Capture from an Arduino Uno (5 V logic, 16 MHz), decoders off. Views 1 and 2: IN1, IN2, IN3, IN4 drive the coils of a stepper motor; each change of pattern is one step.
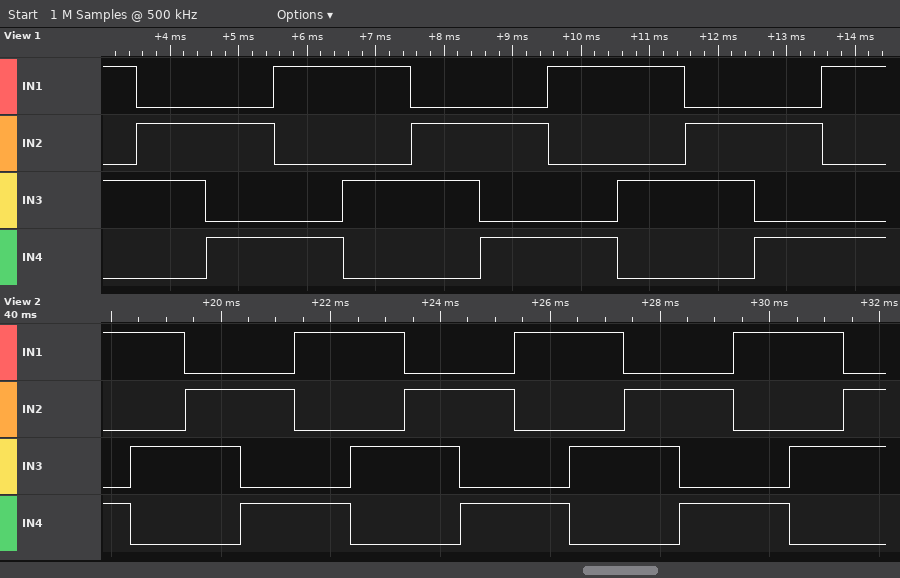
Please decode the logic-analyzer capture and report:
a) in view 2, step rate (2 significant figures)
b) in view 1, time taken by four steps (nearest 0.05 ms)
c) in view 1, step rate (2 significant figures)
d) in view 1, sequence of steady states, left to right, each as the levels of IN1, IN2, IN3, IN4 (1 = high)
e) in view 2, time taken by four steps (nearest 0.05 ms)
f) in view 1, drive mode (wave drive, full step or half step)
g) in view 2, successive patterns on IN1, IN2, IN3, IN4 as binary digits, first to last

1000 steps/s
4.00 ms
1000 steps/s
1010 0110 0101 1001 1010 0110 0101 1001 1010 0110 0101 1001
4.00 ms
full step
1001 1010 0110 0101 1001 1010 0110 0101 1001 1010 0110 0101 1001 1010 0110
